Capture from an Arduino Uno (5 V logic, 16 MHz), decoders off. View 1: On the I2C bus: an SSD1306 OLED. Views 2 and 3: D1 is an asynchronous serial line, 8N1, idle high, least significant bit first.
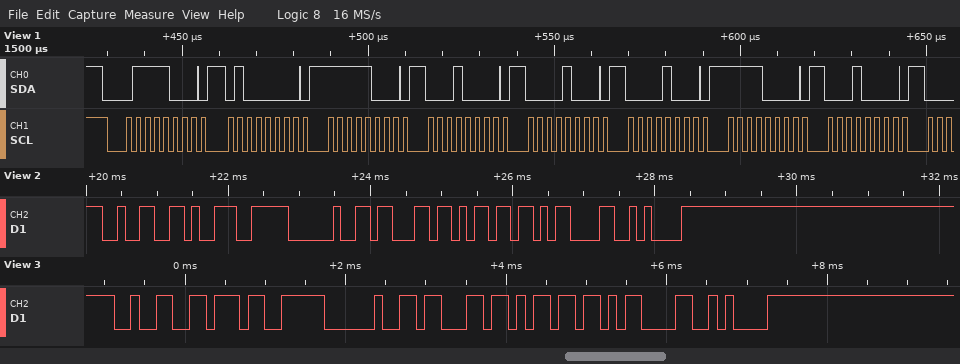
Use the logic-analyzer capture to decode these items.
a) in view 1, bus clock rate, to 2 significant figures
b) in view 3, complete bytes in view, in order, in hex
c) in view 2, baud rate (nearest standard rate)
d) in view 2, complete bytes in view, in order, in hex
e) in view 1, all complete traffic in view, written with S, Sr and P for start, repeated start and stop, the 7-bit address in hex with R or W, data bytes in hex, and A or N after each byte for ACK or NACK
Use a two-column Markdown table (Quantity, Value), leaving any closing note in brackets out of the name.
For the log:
| Quantity | Value |
|---|---|
| in view 1, bus clock rate, to 2 significant figures | 400 kHz |
| in view 3, complete bytes in view, in order, in hex | 32 37 20 63 6D 0D 0A |
| in view 2, baud rate | 9600 baud |
| in view 2, complete bytes in view, in order, in hex | 32 39 20 63 6D 0D 0A |
| in view 1, all complete traffic in view, written with S, Sr and P for start, repeated start and stop, the 7-bit address in hex with R or W, data bytes in hex, and A or N after each byte for ACK or NACK | S 3CW A 40 A F8 A 10 A 08 A 08 A F0 A 10 A |
